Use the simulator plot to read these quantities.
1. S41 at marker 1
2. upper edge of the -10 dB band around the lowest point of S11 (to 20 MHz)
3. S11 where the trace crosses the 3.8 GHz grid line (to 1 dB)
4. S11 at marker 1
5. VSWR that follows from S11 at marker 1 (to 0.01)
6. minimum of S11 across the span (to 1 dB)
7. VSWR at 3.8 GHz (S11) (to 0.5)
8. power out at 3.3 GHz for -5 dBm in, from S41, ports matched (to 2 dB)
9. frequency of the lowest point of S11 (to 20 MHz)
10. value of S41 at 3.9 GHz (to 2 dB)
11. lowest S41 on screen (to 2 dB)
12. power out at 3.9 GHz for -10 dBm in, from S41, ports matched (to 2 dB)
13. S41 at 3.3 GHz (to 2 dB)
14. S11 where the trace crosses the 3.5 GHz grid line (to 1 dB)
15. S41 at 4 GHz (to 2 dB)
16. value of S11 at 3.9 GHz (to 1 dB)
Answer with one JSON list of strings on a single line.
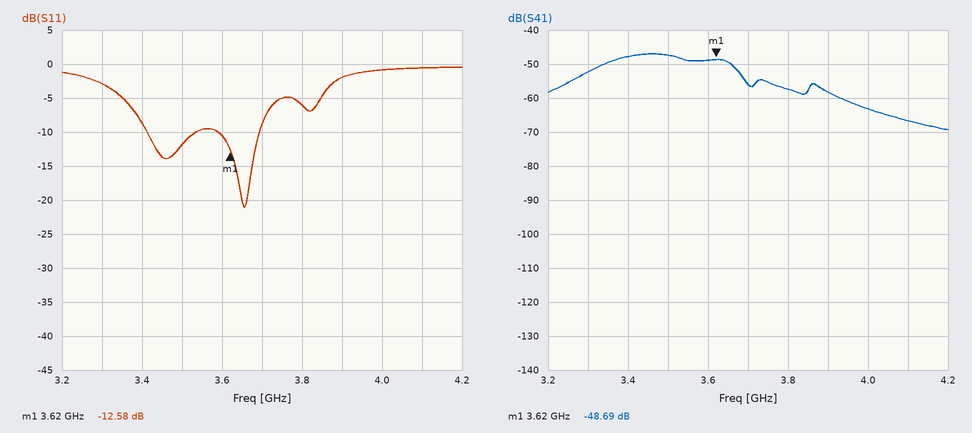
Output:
["-48.69 dB", "3.70 GHz", "-6 dB", "-12.58 dB", "1.61", "-21 dB", "3.0", "-58 dBm", "3.66 GHz", "-58 dB", "-70 dB", "-68 dBm", "-52 dB", "-12 dB", "-64 dB", "-2 dB"]
